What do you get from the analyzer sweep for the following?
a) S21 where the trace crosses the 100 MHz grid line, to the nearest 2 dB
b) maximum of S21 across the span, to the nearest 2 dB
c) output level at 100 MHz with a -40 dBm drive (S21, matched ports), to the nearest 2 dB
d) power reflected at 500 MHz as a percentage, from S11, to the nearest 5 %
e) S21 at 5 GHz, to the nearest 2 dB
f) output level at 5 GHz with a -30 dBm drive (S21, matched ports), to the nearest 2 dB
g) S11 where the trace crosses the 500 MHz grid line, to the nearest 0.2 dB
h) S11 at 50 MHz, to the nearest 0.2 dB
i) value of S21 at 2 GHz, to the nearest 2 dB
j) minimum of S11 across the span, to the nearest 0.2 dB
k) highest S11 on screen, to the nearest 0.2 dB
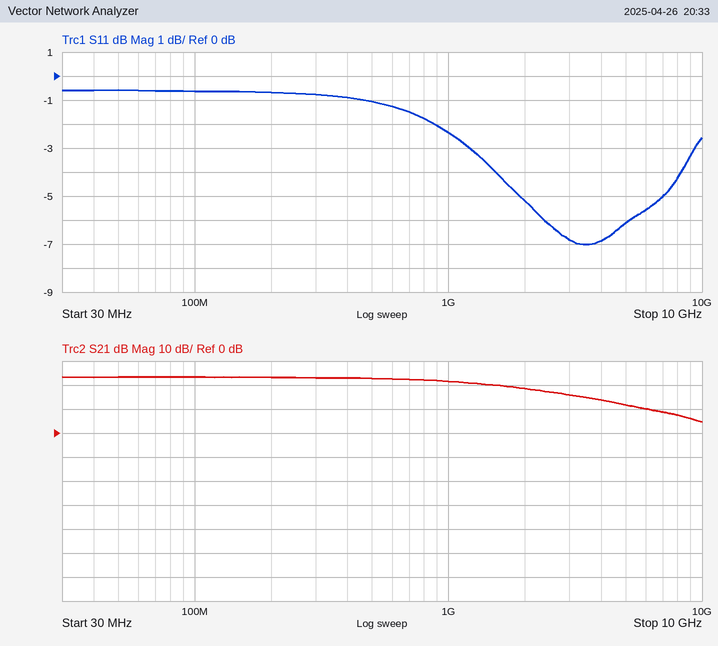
24 dB
24 dB
-16 dBm
80 %
12 dB
-18 dBm
-1.0 dB
-0.6 dB
18 dB
-7.0 dB
-0.6 dB
